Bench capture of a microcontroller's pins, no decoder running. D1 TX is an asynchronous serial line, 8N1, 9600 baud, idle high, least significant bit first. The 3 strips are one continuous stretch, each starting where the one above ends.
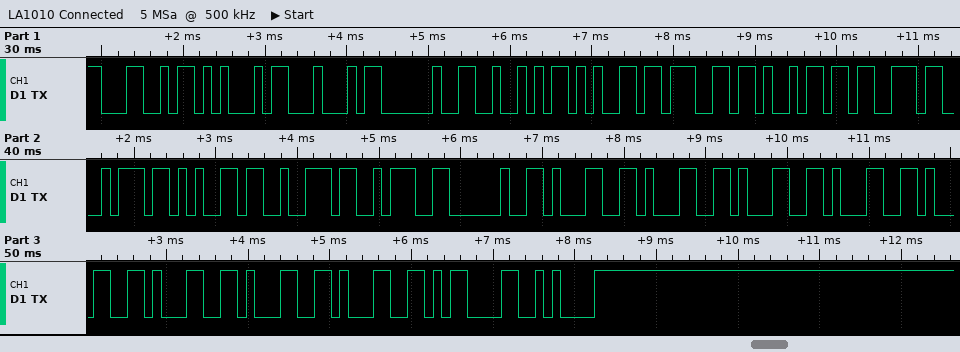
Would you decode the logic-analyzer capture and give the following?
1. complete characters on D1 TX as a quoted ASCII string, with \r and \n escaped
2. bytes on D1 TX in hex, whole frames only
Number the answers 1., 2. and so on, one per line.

1. "LED Register: 11111111\r\n"
2. 0x4C 0x45 0x44 0x20 0x52 0x65 0x67 0x69 0x73 0x74 0x65 0x72 0x3A 0x20 0x31 0x31 0x31 0x31 0x31 0x31 0x31 0x31 0x0D 0x0A
